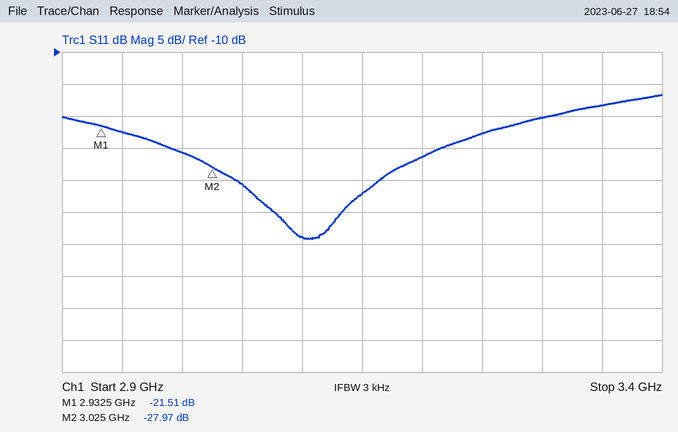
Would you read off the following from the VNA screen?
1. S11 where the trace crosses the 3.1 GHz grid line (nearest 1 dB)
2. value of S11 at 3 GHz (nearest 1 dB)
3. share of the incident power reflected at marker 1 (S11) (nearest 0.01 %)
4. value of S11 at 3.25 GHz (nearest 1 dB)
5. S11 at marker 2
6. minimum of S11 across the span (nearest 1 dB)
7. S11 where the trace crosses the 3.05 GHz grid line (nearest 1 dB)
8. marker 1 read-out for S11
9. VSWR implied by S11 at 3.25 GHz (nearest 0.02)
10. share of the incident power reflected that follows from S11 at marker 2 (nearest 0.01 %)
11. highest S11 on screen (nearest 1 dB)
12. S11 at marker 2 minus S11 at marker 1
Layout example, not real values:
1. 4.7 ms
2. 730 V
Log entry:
1. -39 dB
2. -26 dB
3. 0.71 %
4. -23 dB
5. -27.97 dB
6. -39 dB
7. -31 dB
8. -21.51 dB
9. 1.16
10. 0.16 %
11. -17 dB
12. -6.46 dB
